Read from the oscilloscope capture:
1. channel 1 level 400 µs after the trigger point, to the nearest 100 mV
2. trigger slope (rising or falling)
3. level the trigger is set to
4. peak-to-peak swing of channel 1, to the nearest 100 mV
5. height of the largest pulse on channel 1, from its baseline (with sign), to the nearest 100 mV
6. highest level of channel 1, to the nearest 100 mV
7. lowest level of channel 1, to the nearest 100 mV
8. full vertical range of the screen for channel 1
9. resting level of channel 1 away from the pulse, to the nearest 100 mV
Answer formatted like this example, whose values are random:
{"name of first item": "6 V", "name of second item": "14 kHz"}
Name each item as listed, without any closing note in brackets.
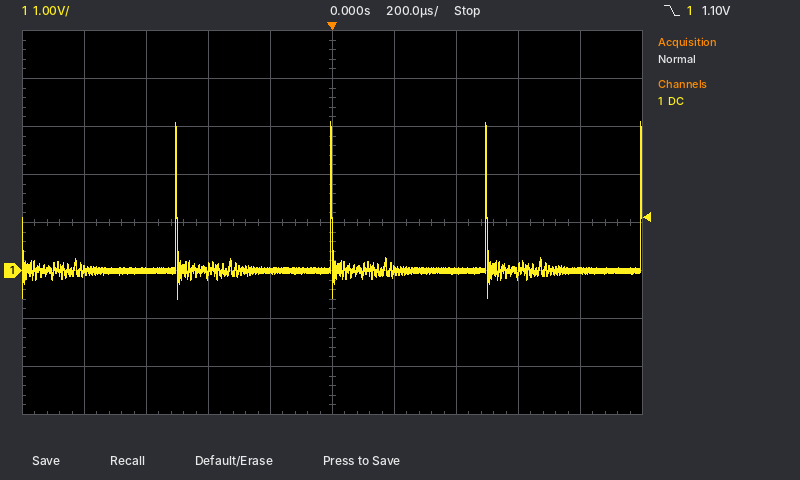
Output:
{"channel 1 level 400 µs after the trigger point, to the nearest 100 mV": "0.0 V", "trigger slope": "falling", "level the trigger is set to": "1.10 V", "peak-to-peak swing of channel 1, to the nearest 100 mV": "3.7 V", "height of the largest pulse on channel 1, from its baseline (with sign), to the nearest 100 mV": "+3.1 V", "highest level of channel 1, to the nearest 100 mV": "3.1 V", "lowest level of channel 1, to the nearest 100 mV": "-600 mV", "full vertical range of the screen for channel 1": "8 V", "resting level of channel 1 away from the pulse, to the nearest 100 mV": "0.0 V"}
